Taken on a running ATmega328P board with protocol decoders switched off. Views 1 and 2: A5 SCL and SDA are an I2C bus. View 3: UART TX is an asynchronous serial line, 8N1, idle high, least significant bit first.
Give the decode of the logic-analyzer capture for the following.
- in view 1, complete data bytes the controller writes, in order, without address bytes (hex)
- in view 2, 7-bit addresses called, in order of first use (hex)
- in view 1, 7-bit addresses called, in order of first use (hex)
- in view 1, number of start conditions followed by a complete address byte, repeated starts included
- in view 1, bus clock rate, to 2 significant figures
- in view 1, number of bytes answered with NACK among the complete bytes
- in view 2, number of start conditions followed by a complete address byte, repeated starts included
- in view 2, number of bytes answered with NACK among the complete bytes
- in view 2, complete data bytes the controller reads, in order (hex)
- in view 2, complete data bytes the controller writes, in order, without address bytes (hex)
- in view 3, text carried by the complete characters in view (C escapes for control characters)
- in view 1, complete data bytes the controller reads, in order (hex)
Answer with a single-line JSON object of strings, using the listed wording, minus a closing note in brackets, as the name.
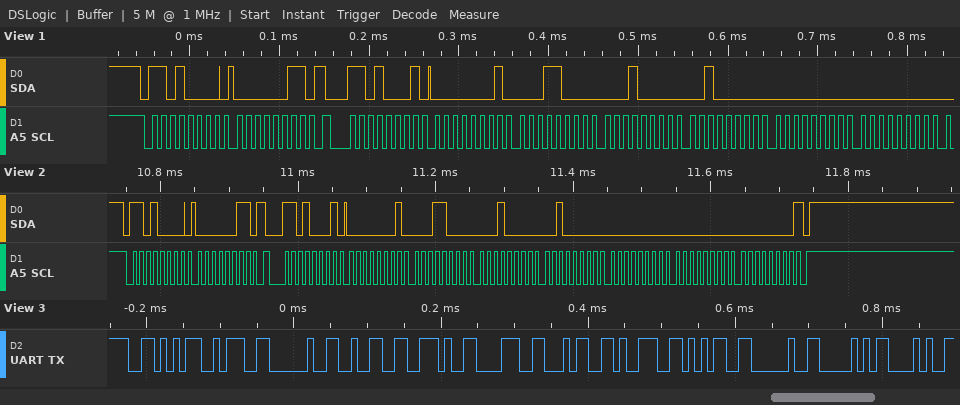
{"in view 1, complete data bytes the controller writes, in order, without address bytes": "03", "in view 2, 7-bit addresses called, in order of first use": "0x68", "in view 1, 7-bit addresses called, in order of first use": "0x68", "in view 1, number of start conditions followed by a complete address byte, repeated starts included": "2", "in view 1, bus clock rate, to 2 significant figures": "100 kHz", "in view 1, number of bytes answered with NACK among the complete bytes": "0", "in view 2, number of start conditions followed by a complete address byte, repeated starts included": "2", "in view 2, number of bytes answered with NACK among the complete bytes": "1", "in view 2, complete data bytes the controller reads, in order": "01 18 10 20 00 00 00", "in view 2, complete data bytes the controller writes, in order, without address bytes": "03", "in view 3, text carried by the complete characters in view": "\"V: 2.8495 P(\"", "in view 1, complete data bytes the controller reads, in order": "01 18 10 20 00 00"}
